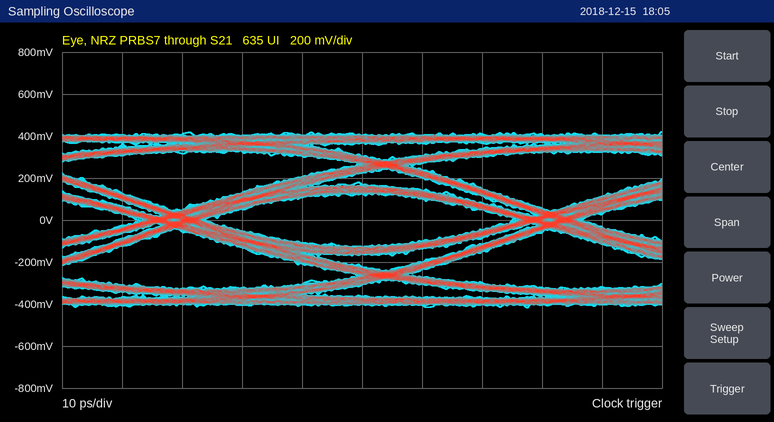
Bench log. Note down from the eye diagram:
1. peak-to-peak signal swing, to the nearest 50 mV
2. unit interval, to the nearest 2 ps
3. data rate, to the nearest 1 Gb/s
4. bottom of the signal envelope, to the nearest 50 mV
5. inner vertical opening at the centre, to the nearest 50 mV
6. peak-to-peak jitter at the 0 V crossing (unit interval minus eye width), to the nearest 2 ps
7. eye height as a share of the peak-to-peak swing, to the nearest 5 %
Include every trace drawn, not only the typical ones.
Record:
850 mV
62 ps
16 Gb/s
-400 mV
250 mV
12 ps
30 %
